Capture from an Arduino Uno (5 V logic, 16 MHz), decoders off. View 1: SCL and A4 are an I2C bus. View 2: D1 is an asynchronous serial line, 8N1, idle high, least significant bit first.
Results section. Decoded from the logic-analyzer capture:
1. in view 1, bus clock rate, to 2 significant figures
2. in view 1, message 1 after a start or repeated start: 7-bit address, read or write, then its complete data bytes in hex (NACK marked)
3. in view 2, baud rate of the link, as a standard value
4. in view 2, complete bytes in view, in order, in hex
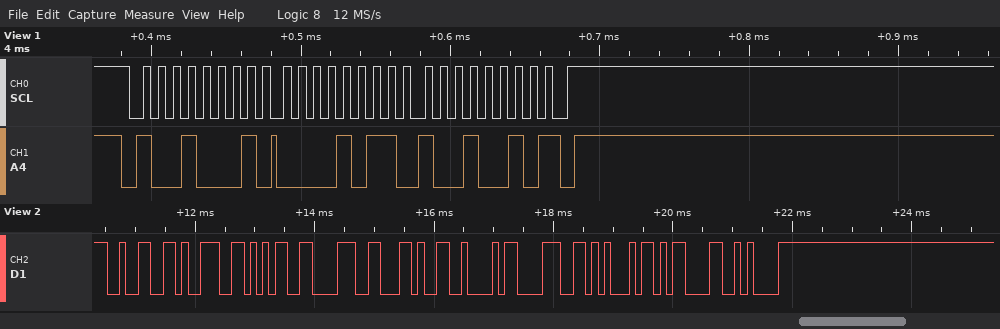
100 kHz
0x48 read: 0B 92 NACK
9600 baud
32 39 35 38 2C 42 38 45 0D 0A
